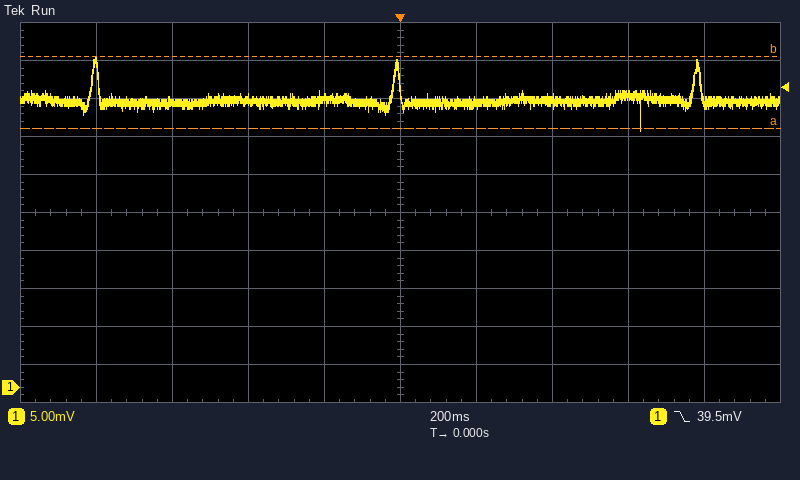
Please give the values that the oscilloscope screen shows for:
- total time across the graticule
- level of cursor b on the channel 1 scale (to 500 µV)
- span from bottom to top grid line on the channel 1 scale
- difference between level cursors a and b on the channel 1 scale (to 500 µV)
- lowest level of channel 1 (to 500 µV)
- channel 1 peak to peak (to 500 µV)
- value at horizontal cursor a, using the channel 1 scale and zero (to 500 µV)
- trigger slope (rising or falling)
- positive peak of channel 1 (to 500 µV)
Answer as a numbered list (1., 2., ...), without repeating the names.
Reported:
1. 2 s
2. 43.5 mV
3. 50 mV
4. 9.5 mV
5. 34.0 mV
6. 9.5 mV
7. 34.0 mV
8. falling
9. 43.5 mV
